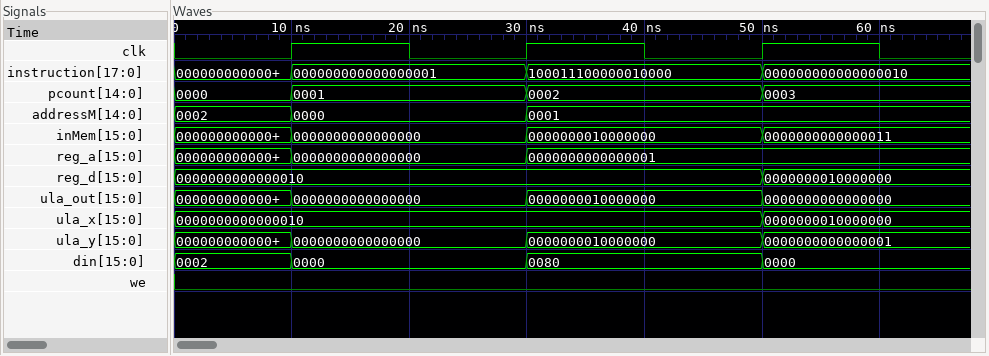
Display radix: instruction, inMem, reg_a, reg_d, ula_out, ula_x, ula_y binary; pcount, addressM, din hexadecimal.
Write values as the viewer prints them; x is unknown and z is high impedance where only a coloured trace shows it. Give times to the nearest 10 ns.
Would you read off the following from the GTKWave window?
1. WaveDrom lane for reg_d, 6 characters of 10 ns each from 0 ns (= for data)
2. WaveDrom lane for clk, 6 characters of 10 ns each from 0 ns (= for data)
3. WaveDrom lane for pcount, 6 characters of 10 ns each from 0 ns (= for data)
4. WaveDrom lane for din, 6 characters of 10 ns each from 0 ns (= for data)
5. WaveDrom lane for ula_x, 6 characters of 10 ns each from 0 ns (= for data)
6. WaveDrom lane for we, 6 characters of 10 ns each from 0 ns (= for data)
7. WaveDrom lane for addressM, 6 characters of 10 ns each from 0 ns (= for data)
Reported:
{name: 'reg_d', wave: '=....=', data: '0000000000000010 0000000010000000'}
{name: 'clk', wave: '010101'}
{name: 'pcount', wave: '==.=.=', data: '0000 0001 0002 0003'}
{name: 'din', wave: '==.=.=', data: '0002 0000 0080 0000'}
{name: 'ula_x', wave: '=....=', data: '0000000000000010 0000000010000000'}
{name: 'we', wave: '0.....'}
{name: 'addressM', wave: '==.=..', data: '0002 0000 0001'}
